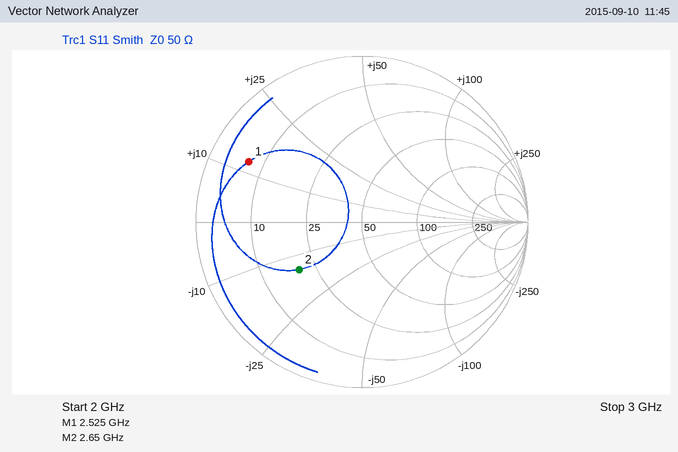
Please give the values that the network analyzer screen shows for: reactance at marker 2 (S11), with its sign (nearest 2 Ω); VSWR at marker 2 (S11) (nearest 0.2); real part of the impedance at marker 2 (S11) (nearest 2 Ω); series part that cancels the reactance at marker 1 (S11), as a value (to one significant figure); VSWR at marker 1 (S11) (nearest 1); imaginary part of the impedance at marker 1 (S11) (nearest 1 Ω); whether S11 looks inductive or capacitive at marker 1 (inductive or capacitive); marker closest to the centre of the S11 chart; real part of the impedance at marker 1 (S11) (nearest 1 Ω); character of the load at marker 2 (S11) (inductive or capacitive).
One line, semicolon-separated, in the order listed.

-14 Ω; 2.8; 20 Ω; 5 pF; 8; +12 Ω; inductive; marker 2; 7 Ω; capacitive
